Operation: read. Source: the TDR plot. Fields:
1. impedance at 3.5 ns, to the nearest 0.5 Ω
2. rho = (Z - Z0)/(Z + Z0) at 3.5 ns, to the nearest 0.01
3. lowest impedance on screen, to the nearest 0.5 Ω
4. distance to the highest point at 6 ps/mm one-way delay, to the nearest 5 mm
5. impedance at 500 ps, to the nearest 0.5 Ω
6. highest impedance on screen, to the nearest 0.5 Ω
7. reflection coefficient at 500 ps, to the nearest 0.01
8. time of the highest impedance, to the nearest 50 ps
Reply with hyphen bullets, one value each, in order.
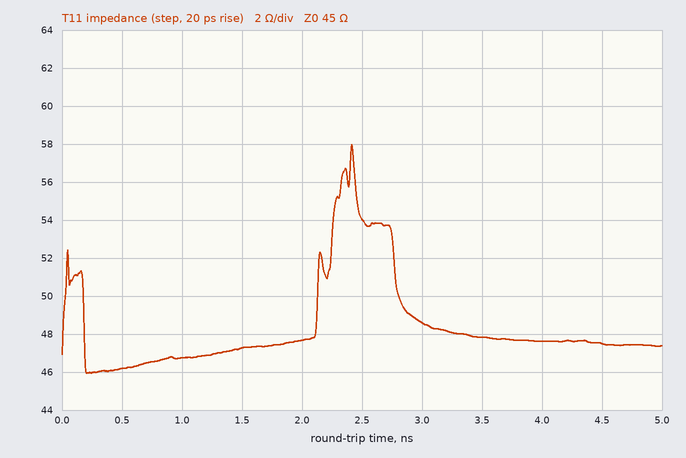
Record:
- 48.0 Ω
- +0.03
- 46.0 Ω
- 200 mm
- 46.0 Ω
- 58.0 Ω
- +0.01
- 2.40 ns
